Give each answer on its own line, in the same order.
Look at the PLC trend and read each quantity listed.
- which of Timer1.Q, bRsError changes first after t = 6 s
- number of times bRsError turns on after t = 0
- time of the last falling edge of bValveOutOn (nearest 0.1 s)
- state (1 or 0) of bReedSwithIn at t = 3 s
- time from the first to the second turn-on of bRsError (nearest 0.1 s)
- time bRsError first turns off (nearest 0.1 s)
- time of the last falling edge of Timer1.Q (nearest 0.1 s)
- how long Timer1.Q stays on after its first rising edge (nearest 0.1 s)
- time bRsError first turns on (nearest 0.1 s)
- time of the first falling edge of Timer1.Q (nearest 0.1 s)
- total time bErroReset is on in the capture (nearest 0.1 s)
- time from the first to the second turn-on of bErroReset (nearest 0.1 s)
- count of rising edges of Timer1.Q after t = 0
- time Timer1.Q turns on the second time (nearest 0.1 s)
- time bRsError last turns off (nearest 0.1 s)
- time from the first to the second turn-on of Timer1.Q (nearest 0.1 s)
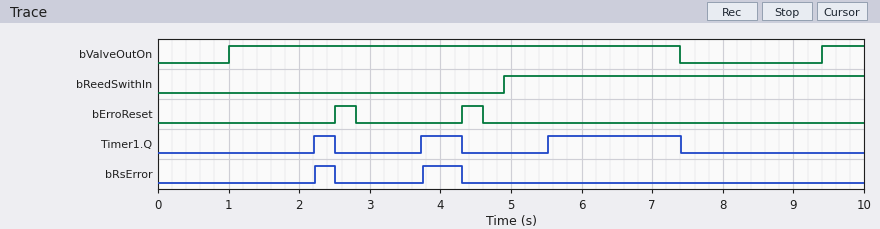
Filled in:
Timer1.Q
2
7.4 s
0
1.5 s
2.5 s
7.4 s
0.3 s
2.2 s
2.5 s
0.6 s
1.8 s
3
3.7 s
4.3 s
1.5 s
